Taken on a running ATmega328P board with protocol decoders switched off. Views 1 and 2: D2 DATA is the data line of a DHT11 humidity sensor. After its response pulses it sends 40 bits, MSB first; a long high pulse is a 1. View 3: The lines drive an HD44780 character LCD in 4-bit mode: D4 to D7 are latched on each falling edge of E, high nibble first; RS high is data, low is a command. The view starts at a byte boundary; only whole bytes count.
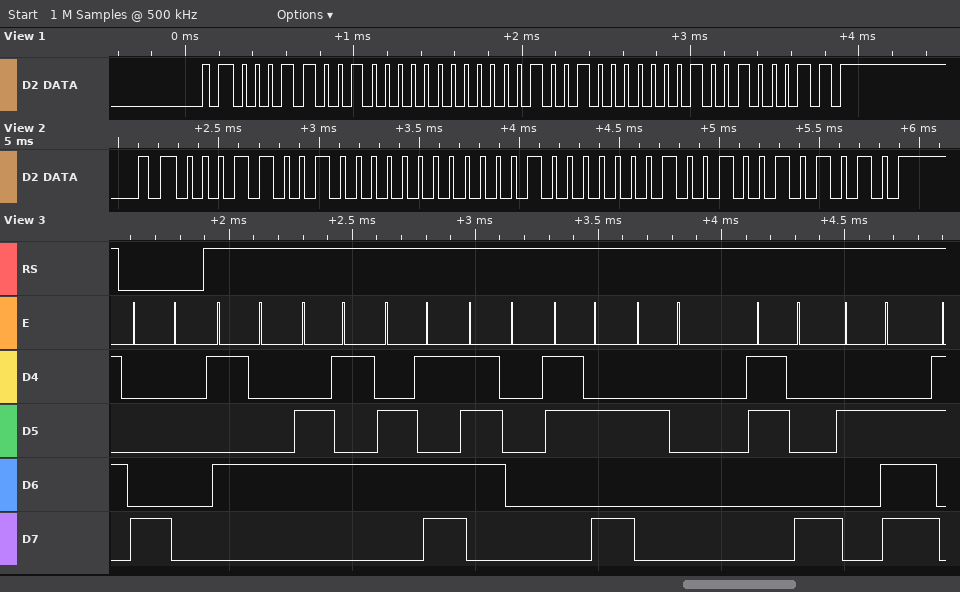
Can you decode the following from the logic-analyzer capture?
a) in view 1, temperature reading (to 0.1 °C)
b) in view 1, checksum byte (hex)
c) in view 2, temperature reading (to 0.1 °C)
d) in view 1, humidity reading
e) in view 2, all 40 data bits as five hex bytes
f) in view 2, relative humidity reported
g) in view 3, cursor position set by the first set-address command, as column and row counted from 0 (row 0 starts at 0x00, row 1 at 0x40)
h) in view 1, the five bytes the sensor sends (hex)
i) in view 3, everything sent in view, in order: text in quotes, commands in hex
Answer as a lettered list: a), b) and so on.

a) 9.1 °C
b) 0x23
c) 8.9 °C
d) 25 %
e) 19 00 08 09 2A
f) 25 %
g) column 0, row 0
h) 19 00 09 01 23
i) 0x80 "Temp: 8."
